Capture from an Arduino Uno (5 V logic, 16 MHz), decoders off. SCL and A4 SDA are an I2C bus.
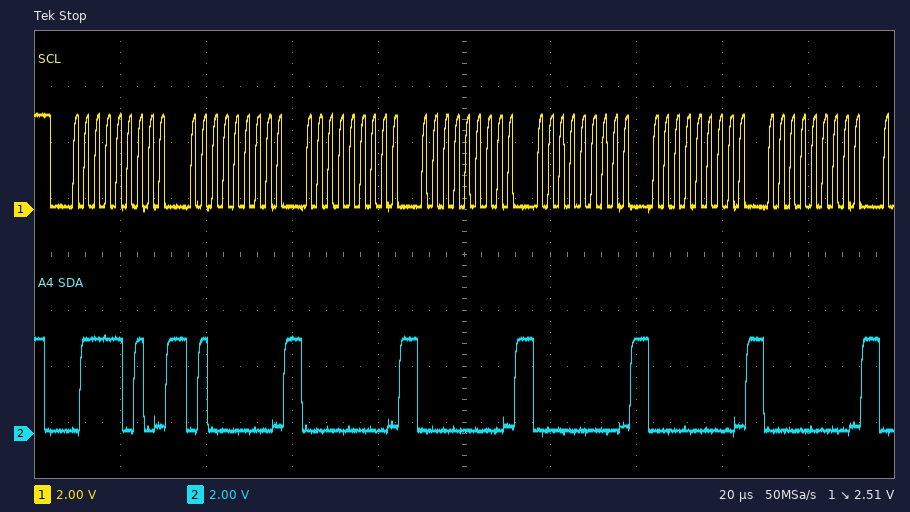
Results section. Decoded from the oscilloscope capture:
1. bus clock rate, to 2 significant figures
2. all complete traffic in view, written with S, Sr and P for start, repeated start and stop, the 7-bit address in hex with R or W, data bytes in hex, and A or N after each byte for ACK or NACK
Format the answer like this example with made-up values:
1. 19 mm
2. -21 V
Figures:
1. 400 kHz
2. S 3DW A 40 A 00 A 00 A 00 A 00 A 00 A
